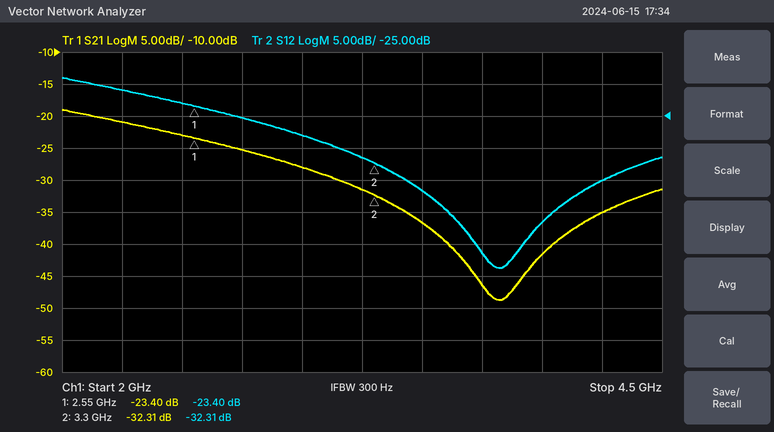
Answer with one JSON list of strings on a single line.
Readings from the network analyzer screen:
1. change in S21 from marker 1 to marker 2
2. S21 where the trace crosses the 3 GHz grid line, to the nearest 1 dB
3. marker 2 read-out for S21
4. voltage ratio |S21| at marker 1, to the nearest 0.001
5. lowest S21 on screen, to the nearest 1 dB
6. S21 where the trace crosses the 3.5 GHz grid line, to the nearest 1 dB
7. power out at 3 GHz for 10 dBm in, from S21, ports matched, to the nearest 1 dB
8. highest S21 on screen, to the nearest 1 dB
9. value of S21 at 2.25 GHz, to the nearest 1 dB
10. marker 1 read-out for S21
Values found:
["-8.91 dB", "-28 dB", "-32.31 dB", "0.068", "-49 dB", "-37 dB", "-18 dBm", "-19 dB", "-21 dB", "-23.40 dB"]
